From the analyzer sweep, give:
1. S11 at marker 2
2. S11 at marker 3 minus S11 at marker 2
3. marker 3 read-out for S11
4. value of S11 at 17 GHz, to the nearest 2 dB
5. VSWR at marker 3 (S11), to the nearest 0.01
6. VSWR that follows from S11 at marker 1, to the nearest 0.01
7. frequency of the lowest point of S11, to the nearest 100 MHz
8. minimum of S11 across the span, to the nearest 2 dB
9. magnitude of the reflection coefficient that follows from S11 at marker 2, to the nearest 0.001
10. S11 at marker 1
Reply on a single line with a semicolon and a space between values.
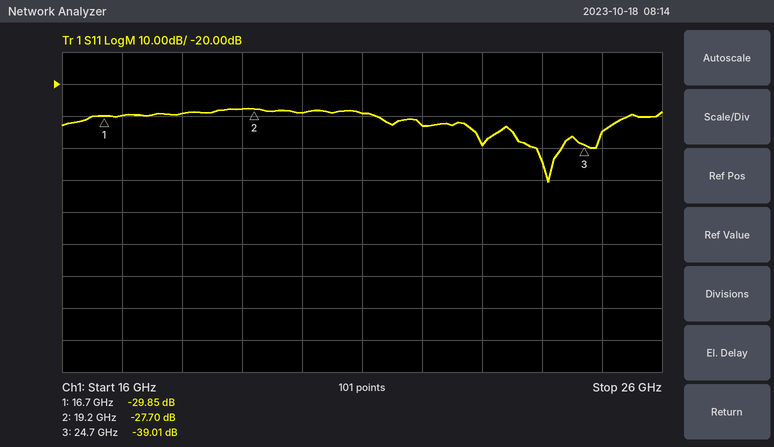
-27.70 dB; -11.31 dB; -39.01 dB; -30 dB; 1.02; 1.07; 24.1 GHz; -50 dB; 0.041; -29.85 dB
